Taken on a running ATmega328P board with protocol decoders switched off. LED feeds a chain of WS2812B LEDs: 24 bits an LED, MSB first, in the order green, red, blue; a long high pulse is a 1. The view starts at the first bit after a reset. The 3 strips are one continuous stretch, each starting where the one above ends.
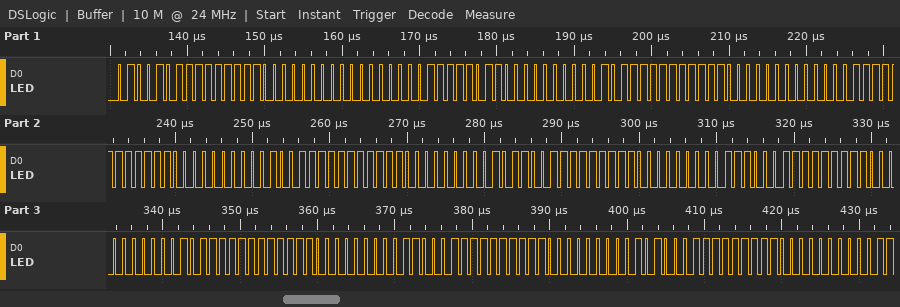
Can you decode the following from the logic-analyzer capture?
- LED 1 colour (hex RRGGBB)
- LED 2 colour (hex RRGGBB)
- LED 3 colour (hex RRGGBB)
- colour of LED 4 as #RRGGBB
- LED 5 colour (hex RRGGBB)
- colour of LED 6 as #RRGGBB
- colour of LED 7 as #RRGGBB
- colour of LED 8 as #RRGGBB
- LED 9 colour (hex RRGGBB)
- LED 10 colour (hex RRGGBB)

#FE4B00
#FB0000
#FE2F00
#FE0F00
#FE4F00
#FEB300
#FEE300
#FE5F00
#FEC700
#FEA300
